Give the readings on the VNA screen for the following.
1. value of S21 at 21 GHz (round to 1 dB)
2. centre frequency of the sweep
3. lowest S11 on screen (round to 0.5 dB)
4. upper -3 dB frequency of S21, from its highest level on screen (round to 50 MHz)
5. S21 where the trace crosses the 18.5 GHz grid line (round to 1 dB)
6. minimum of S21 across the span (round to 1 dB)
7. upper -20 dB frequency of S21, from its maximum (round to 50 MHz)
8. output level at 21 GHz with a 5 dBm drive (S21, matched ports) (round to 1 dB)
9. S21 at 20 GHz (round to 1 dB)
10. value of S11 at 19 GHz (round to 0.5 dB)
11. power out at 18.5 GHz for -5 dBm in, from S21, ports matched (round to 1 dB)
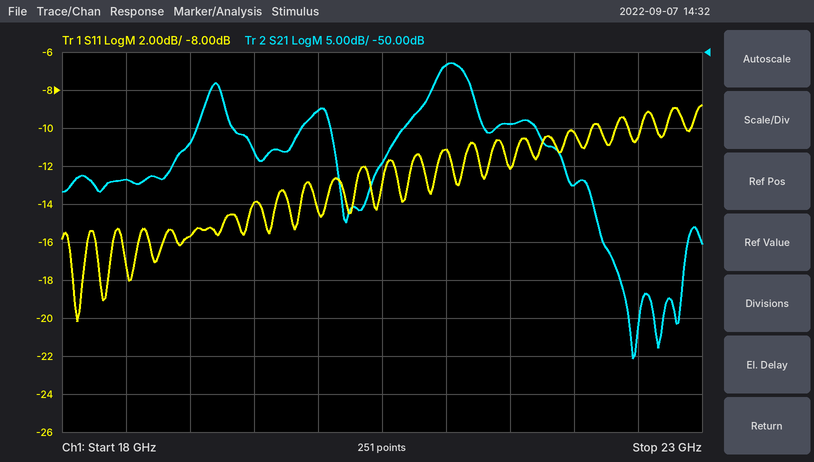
-52 dB
20.5 GHz
-20.0 dB
21.20 GHz
-67 dB
-90 dB
22.15 GHz
-47 dBm
-58 dB
-15.5 dB
-72 dBm
